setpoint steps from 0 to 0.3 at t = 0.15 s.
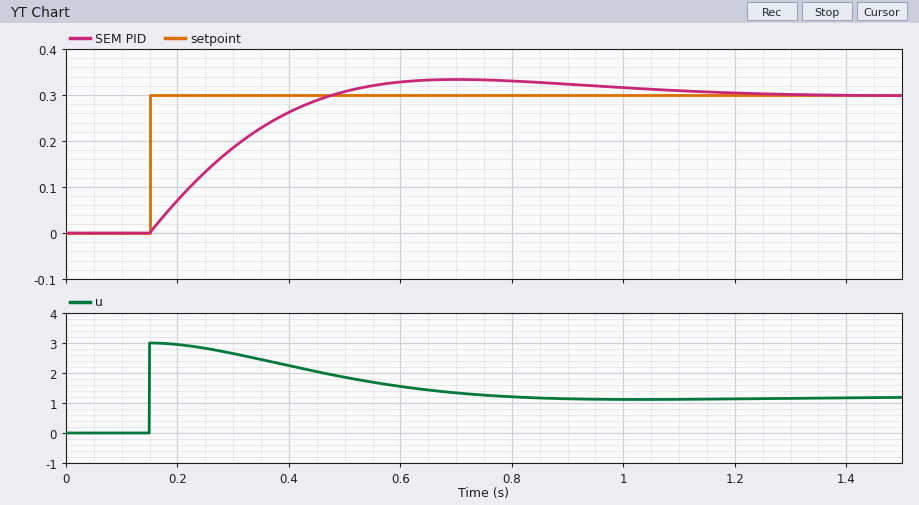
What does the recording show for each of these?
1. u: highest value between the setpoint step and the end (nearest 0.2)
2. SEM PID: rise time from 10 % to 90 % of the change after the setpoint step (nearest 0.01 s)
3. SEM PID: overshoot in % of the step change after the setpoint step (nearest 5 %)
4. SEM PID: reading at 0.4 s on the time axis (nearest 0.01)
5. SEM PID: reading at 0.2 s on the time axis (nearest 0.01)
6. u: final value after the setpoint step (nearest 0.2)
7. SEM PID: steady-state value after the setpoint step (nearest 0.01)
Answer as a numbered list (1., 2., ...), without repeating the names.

1. 3.0
2. 0.24 s
3. 10 %
4. 0.26
5. 0.07
6. 1.2
7. 0.30
